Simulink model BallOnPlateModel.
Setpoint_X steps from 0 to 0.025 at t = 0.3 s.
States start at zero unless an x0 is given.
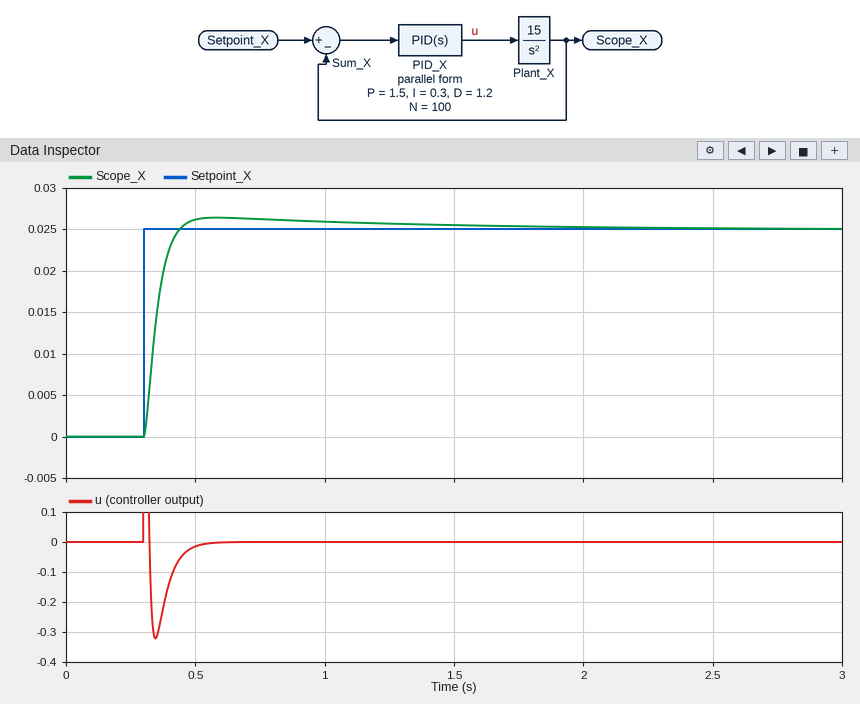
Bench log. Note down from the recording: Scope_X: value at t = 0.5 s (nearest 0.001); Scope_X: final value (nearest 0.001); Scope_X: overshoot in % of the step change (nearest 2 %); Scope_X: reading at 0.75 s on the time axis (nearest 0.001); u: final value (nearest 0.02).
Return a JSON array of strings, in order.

["0.026", "0.025", "6 %", "0.026", "0.00"]
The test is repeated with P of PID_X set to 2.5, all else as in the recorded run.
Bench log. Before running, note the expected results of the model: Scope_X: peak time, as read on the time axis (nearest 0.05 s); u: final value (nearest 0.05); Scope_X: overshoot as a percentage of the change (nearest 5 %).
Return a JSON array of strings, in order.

["0.55 s", "0.00", "10 %"]
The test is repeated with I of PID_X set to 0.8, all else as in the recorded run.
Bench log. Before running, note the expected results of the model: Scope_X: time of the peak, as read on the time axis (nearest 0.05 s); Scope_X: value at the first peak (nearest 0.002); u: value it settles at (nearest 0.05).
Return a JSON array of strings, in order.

["0.60 s", "0.026", "0.00"]
